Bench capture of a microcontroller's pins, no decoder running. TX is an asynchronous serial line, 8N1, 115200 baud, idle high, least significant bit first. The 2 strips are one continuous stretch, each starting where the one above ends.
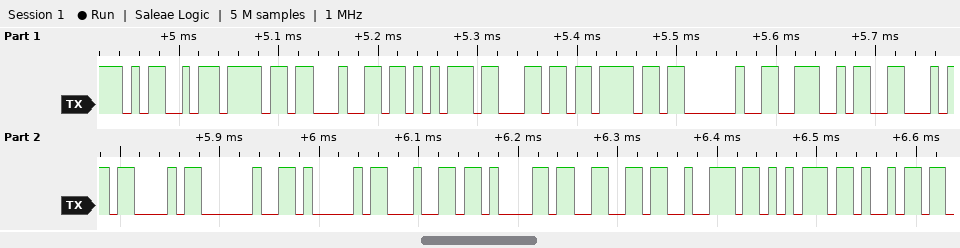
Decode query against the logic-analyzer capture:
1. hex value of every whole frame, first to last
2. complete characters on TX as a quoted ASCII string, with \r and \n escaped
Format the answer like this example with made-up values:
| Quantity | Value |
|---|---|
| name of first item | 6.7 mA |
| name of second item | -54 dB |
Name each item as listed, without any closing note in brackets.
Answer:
| Quantity | Value |
|---|---|
| hex value of every whole frame, first to last | 0x4D 0x6F 0x64 0x75 0x6C 0x6F 0x20 0x4E 0x46 0x43 0x20 0x41 0x64 0x61 0x66 0x72 0x75 0x69 |
| complete characters on TX as a quoted ASCII string, with \r and \n escaped | "Modulo NFC Adafrui" |
